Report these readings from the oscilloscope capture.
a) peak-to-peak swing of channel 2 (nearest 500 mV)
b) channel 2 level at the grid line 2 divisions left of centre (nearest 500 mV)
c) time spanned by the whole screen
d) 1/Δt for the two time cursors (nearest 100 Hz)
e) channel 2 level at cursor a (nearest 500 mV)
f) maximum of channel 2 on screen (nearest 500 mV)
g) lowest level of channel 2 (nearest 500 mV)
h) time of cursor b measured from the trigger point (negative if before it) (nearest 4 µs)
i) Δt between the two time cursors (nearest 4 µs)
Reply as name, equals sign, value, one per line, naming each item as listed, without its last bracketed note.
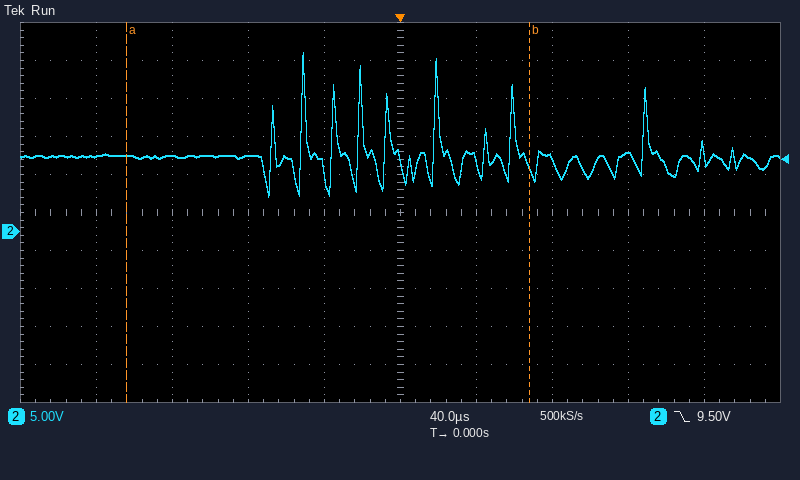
peak-to-peak swing of channel 2 = 19.0 V
channel 2 level at the grid line 2 divisions left of centre = 10.0 V
time spanned by the whole screen = 400 µs
1/Δt for the two time cursors = 4.7 kHz
channel 2 level at cursor a = 10.0 V
maximum of channel 2 on screen = 23.5 V
lowest level of channel 2 = 4.5 V
time of cursor b measured from the trigger point (negative if before it) = +68 µs
Δt between the two time cursors = 212 µs
